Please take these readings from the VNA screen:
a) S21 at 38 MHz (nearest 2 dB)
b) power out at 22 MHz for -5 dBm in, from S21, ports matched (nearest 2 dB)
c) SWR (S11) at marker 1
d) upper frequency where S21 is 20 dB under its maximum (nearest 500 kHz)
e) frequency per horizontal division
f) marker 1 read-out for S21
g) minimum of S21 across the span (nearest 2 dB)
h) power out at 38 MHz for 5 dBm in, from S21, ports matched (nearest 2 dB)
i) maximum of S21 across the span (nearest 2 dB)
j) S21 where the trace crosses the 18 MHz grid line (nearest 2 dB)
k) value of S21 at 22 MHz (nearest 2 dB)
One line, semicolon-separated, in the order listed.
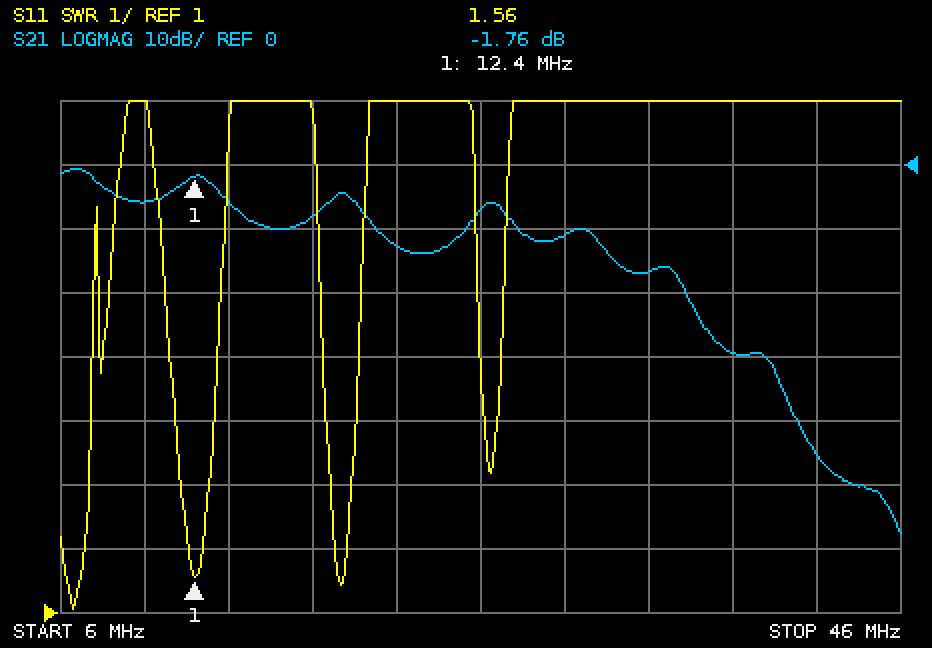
-30 dB; -18 dBm; 1.56; 36.0 MHz; 4 MHz; -1.76 dB; -58 dB; -24 dBm; 0 dB; -8 dB; -12 dB
